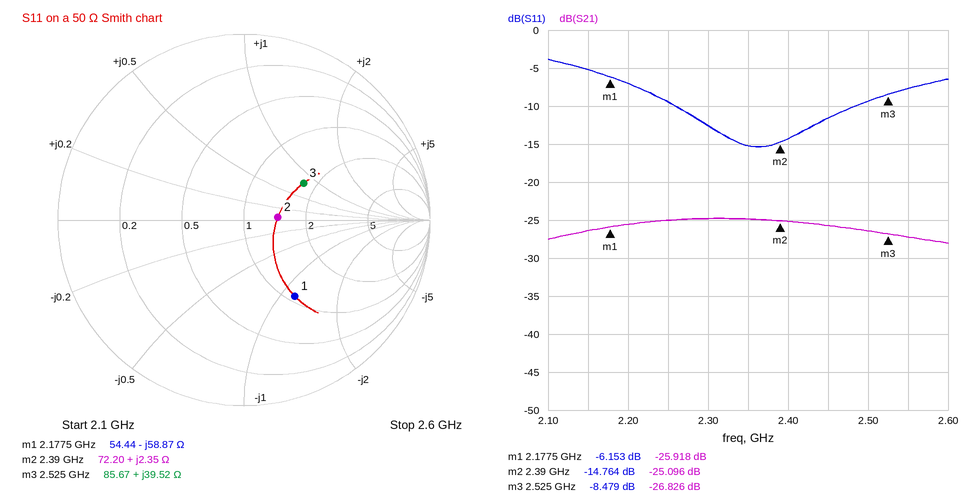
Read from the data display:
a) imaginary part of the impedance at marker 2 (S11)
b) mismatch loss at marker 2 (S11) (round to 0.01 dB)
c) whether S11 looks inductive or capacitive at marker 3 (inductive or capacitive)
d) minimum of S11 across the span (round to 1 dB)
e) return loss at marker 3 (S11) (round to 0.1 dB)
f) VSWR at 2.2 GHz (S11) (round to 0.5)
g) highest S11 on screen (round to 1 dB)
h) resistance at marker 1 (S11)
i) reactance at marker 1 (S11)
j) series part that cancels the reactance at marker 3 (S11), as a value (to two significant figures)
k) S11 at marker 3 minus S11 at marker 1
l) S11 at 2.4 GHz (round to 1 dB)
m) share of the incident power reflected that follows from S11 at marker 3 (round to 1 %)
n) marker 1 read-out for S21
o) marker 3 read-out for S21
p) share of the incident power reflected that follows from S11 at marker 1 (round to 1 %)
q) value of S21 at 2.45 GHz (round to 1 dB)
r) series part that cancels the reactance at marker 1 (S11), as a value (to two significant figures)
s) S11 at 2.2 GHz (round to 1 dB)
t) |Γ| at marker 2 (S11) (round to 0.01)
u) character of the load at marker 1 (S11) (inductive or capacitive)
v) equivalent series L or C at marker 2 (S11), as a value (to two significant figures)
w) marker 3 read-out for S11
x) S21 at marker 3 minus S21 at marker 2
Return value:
+2.35 Ω
0.15 dB
inductive
-15 dB
8.5 dB
2.5
-4 dB
54.44 Ω
-58.87 Ω
1.6 pF
-2.326 dB
-14 dB
14 %
-25.918 dB
-26.826 dB
24 %
-26 dB
4.3 nH
-7 dB
0.18
capacitive
160 pH
-8.479 dB
-1.730 dB
